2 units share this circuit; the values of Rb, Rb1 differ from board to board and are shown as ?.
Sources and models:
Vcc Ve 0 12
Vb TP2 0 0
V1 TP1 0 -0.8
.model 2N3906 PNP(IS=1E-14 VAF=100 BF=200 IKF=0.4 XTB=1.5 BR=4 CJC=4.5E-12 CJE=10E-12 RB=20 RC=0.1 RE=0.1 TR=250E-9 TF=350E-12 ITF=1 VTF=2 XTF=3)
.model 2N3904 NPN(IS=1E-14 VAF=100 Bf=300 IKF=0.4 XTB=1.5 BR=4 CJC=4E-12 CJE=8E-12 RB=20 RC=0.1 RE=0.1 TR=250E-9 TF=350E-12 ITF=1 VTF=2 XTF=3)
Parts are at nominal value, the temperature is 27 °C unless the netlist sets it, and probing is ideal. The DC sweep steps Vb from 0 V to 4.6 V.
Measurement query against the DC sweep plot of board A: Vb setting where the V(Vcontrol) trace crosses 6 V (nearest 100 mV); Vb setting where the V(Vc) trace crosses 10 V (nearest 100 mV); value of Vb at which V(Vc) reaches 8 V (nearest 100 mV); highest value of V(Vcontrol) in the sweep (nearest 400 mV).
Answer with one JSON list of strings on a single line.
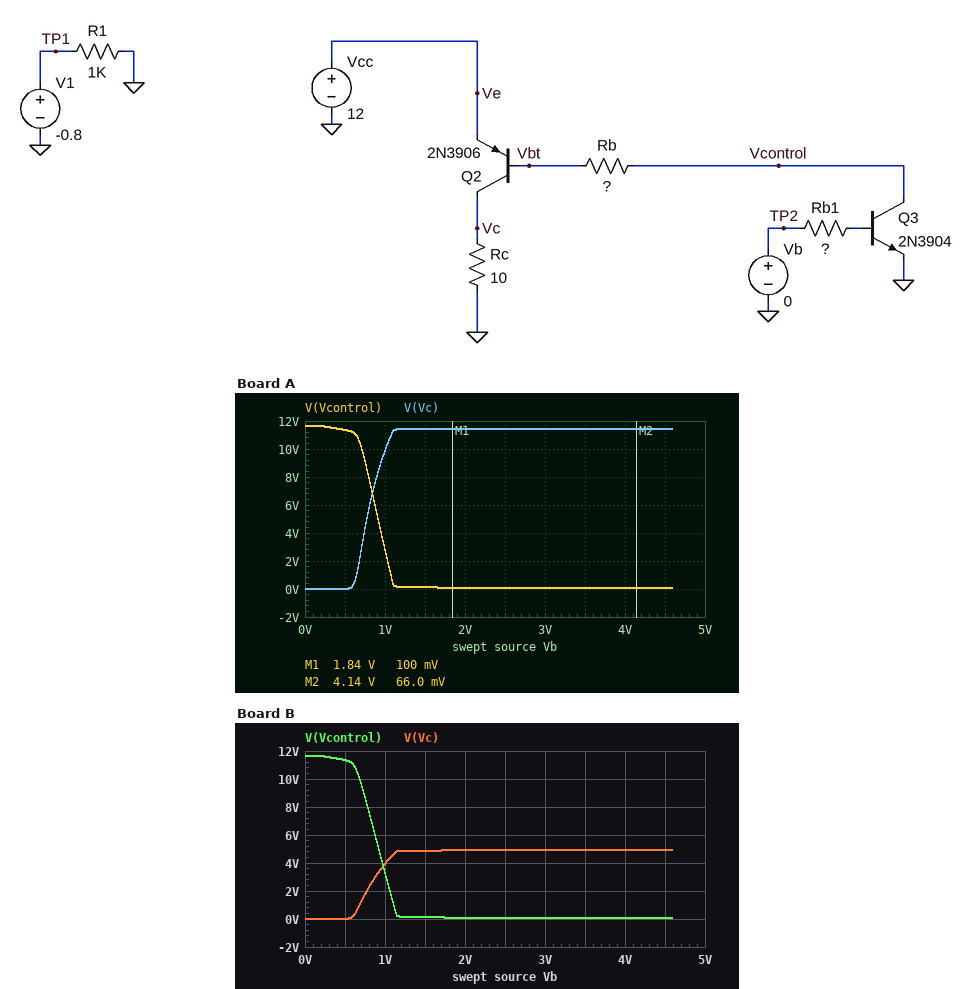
["900 mV", "1.0 V", "900 mV", "11.6 V"]
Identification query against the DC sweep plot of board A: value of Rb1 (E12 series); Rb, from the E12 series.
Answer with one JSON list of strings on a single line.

["4.7 kΩ", "470 Ω"]
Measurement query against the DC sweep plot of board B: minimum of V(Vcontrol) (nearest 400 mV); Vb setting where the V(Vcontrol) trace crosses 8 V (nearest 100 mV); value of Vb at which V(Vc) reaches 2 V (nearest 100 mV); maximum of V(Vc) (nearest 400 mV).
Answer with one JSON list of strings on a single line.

["0 V", "800 mV", "800 mV", "4.8 V"]
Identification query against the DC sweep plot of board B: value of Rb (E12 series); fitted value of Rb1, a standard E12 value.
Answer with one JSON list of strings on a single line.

["2.2 kΩ", "27 kΩ"]
